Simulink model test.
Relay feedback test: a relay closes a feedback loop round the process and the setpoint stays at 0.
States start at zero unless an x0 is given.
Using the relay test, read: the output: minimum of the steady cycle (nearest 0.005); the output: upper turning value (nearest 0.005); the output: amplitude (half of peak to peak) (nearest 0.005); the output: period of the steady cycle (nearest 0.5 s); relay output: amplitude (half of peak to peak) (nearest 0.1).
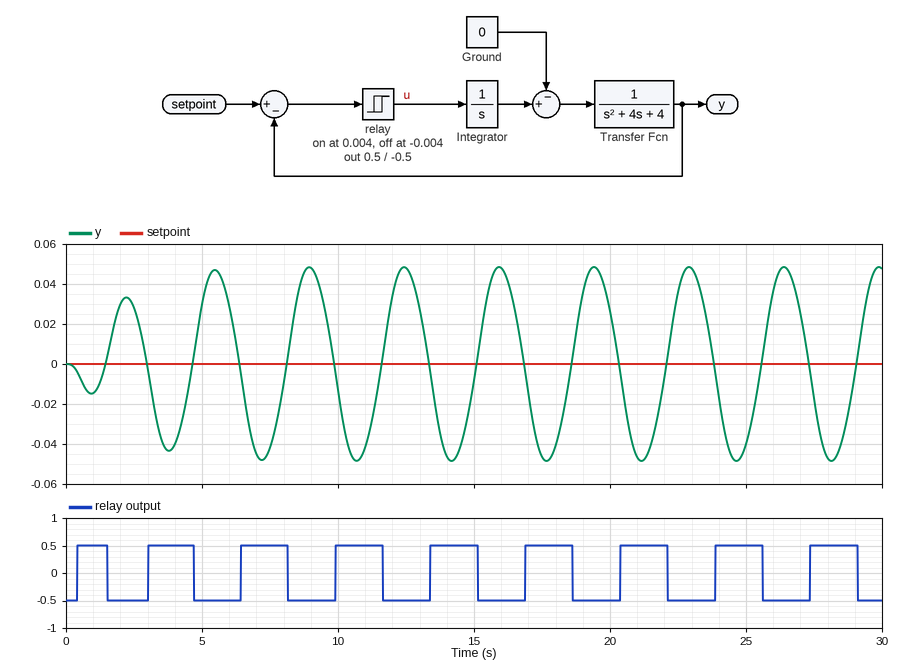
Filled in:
-0.050
0.050
0.050
3.5 s
0.5
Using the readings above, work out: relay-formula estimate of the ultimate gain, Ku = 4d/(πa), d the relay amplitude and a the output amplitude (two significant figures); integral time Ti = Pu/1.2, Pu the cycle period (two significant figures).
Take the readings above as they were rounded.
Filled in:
13
2.9 s
